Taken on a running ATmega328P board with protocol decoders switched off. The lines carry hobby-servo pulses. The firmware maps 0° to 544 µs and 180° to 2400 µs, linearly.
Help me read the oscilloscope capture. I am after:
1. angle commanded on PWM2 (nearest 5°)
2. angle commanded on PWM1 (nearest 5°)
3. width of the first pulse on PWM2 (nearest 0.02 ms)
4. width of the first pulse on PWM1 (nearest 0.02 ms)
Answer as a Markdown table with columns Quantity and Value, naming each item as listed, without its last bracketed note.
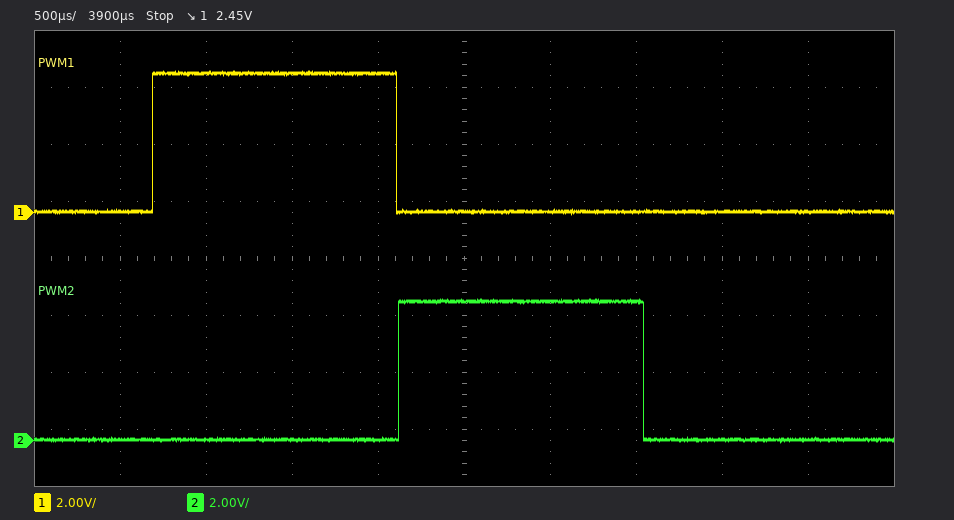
| Quantity | Value |
|---|---|
| angle commanded on PWM2 | 85° |
| angle commanded on PWM1 | 85° |
| width of the first pulse on PWM2 | 1.42 ms |
| width of the first pulse on PWM1 | 1.42 ms |
